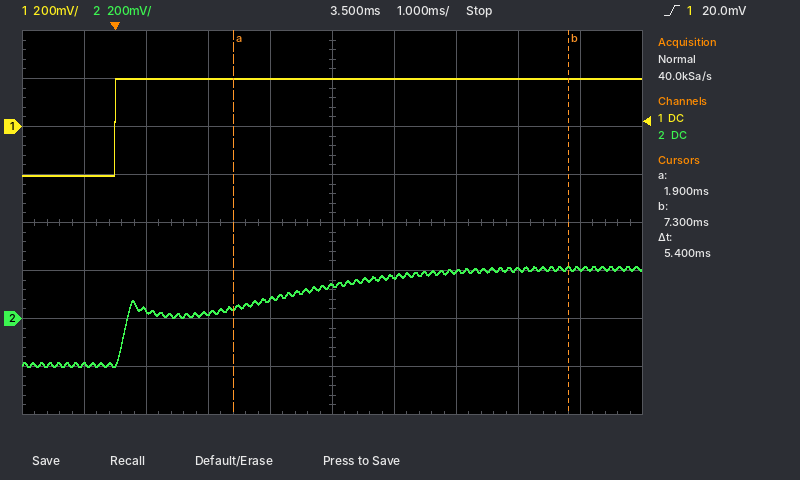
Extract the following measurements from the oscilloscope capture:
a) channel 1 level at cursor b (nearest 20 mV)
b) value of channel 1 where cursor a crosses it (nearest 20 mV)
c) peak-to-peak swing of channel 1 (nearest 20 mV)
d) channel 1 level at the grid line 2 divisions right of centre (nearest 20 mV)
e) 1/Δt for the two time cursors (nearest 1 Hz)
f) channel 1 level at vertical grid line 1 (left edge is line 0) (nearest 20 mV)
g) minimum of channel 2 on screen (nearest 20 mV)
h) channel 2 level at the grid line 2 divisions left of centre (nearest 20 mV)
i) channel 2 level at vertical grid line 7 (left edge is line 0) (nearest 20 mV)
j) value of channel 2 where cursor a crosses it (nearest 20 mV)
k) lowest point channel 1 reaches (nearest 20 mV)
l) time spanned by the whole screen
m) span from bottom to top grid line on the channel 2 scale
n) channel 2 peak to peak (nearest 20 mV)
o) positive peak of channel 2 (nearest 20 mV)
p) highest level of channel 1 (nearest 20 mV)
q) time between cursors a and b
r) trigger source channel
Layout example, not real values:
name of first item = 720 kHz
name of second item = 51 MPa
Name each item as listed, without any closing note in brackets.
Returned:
channel 1 level at cursor b = 200 mV
value of channel 1 where cursor a crosses it = 200 mV
peak-to-peak swing of channel 1 = 400 mV
channel 1 level at the grid line 2 divisions right of centre = 200 mV
1/Δt for the two time cursors = 185 Hz
channel 1 level at vertical grid line 1 (left edge is line 0) = -200 mV
minimum of channel 2 on screen = -200 mV
channel 2 level at the grid line 2 divisions left of centre = 20 mV
channel 2 level at vertical grid line 7 (left edge is line 0) = 200 mV
value of channel 2 where cursor a crosses it = 40 mV
lowest point channel 1 reaches = -200 mV
time spanned by the whole screen = 10 ms
span from bottom to top grid line on the channel 2 scale = 1.6 V
channel 2 peak to peak = 420 mV
positive peak of channel 2 = 220 mV
highest level of channel 1 = 200 mV
time between cursors a and b = 5.4 ms
trigger source channel = channel 1
